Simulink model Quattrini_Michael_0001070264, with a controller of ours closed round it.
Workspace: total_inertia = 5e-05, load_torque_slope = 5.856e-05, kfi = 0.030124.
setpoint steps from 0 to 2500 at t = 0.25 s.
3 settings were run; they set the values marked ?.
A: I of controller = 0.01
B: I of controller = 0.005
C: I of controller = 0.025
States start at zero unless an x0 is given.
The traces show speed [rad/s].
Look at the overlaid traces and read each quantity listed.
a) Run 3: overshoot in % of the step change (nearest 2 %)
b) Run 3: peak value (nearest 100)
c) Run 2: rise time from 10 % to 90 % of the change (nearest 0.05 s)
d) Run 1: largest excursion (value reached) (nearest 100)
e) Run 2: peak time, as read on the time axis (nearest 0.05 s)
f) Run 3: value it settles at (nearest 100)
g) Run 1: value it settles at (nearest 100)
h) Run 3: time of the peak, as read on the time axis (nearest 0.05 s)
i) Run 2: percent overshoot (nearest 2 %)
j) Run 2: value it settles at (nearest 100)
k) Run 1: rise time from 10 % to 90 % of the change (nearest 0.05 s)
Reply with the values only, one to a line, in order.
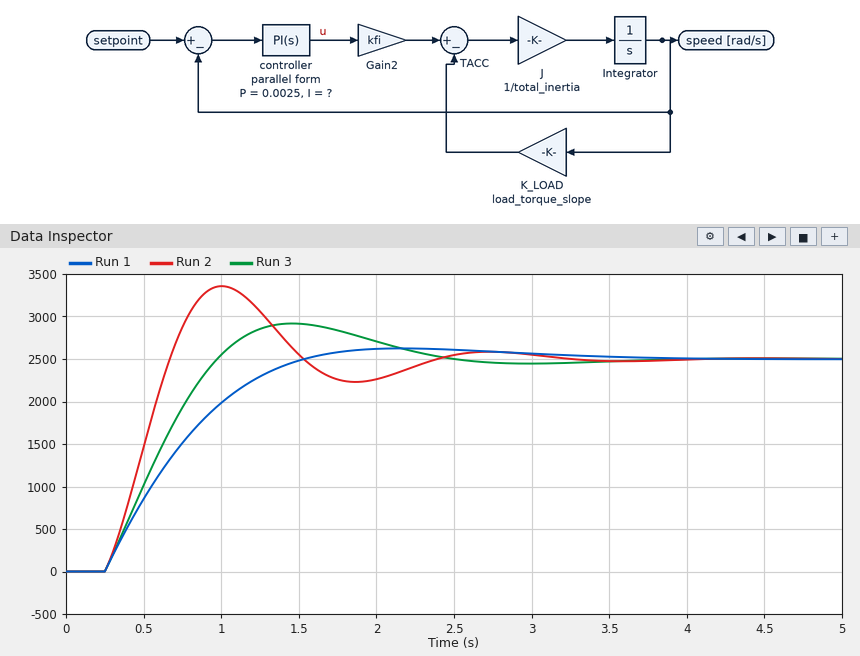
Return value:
16 %
2900
0.30 s
2600
1.00 s
2500
2500
1.45 s
34 %
2500
0.90 s
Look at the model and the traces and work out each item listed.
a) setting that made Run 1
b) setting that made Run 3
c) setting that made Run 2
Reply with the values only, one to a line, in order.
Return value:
B
A
C
